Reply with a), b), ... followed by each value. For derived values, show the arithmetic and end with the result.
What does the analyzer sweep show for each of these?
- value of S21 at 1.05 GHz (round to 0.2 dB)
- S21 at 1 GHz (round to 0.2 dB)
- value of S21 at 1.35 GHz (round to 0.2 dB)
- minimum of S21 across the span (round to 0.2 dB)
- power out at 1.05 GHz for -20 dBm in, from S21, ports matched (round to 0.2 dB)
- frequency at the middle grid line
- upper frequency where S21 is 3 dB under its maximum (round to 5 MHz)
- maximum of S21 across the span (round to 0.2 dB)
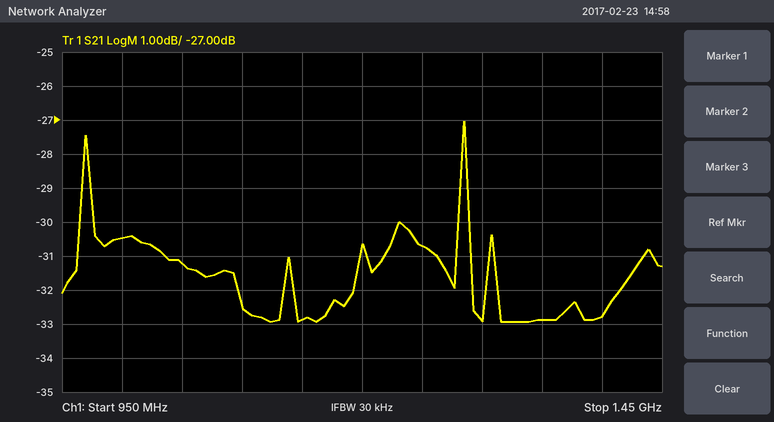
a) -31.2 dB
b) -30.4 dB
c) -32.8 dB
d) -33.0 dB
e) -20 dBm + (-31.2 dB) = -51.2 dBm
f) 1.2 GHz
g) 1.290 GHz
h) -27.0 dB
